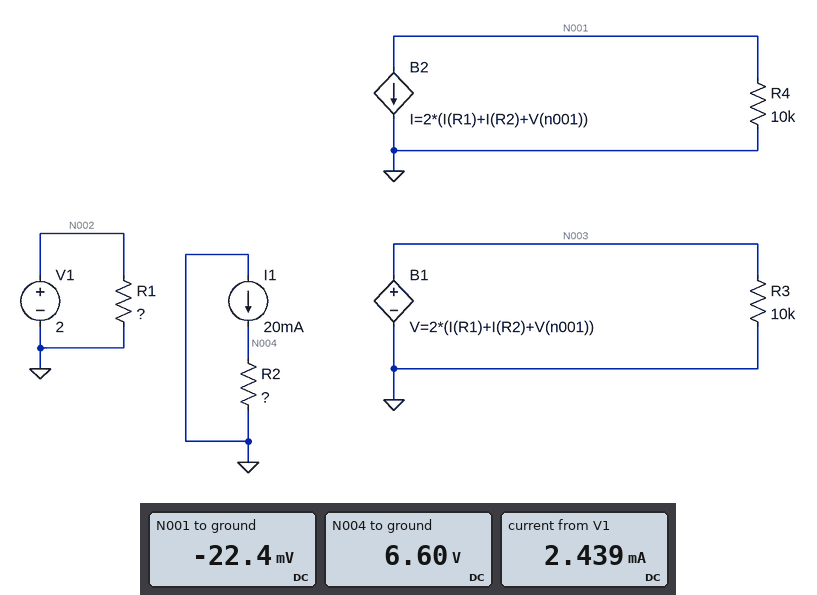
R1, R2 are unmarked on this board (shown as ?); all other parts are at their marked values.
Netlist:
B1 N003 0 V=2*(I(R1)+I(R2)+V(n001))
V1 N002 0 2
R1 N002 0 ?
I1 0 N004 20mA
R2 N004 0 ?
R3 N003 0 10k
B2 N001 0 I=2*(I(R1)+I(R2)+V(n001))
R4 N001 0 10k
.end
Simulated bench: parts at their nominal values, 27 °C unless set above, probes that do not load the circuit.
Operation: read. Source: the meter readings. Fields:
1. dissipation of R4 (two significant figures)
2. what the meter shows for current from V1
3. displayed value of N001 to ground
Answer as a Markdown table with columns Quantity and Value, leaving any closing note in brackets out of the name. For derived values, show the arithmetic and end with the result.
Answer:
| Quantity | Value |
|---|---|
| dissipation of R4 | (0 V - (-22.4 mV))^2 / 10 kΩ = 50 nW |
| what the meter shows for current from V1 | 2.439 mA |
| displayed value of N001 to ground | -22.4 mV |
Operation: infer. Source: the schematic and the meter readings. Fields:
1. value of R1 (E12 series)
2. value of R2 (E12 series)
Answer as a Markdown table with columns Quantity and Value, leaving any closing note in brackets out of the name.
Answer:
| Quantity | Value |
|---|---|
| value of R1 | 820 Ω |
| value of R2 | 330 Ω |
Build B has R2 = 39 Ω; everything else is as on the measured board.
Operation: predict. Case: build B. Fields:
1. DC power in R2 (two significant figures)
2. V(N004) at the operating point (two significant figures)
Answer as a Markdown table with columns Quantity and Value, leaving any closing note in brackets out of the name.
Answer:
| Quantity | Value |
|---|---|
| DC power in R2 | 16 mW |
| V(N004) at the operating point | 780 mV |
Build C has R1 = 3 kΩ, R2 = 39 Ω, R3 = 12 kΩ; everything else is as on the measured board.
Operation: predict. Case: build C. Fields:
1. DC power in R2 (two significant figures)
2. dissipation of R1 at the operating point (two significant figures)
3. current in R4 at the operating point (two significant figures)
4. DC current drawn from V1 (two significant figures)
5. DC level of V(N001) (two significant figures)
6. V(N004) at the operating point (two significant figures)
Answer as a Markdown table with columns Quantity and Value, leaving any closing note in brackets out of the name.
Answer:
| Quantity | Value |
|---|---|
| DC power in R2 | 16 mW |
| dissipation of R1 at the operating point | 1.3 mW |
| current in R4 at the operating point | 2.1 µA |
| DC current drawn from V1 | 670 µA |
| DC level of V(N001) | -21 mV |
| V(N004) at the operating point | 780 mV |
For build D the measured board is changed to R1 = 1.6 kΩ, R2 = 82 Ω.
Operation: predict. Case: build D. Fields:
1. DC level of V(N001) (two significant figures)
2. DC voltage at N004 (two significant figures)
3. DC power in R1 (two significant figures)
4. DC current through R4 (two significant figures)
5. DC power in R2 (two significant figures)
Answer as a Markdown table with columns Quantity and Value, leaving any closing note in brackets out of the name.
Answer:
| Quantity | Value |
|---|---|
| DC level of V(N001) | -21 mV |
| DC voltage at N004 | 1.6 V |
| DC power in R1 | 2.5 mW |
| DC current through R4 | 2.1 µA |
| DC power in R2 | 33 mW |
